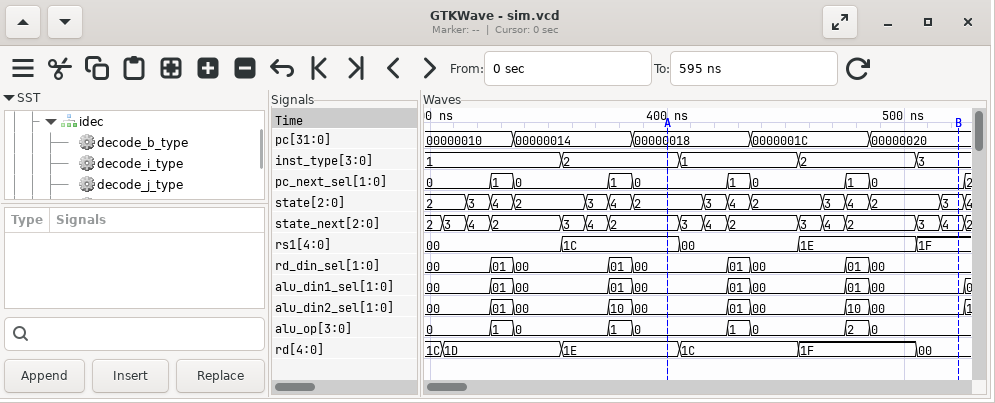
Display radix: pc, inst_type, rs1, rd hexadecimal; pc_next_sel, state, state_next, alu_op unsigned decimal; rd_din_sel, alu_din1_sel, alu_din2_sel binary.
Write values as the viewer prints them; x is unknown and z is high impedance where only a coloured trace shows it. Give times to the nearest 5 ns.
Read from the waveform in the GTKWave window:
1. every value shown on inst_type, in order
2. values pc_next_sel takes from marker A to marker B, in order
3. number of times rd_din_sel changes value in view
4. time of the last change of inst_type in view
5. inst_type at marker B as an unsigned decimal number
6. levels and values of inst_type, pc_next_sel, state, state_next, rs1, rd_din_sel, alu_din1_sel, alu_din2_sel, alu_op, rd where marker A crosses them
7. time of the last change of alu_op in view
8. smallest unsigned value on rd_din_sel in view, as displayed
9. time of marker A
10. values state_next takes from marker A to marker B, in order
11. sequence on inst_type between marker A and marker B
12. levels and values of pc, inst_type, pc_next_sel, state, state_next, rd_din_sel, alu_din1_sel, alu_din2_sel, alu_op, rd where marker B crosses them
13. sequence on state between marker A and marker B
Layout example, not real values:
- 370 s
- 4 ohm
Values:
- 1, 2, 1, 2, 3
- 0, 1, 0, 1, 0
- 8
- 505 ns
- 3
- inst_type=2, pc_next_sel=0, state=2, state_next=2, rs1=1C, rd_din_sel=00, alu_din1_sel=00, alu_din2_sel=00, alu_op=0, rd=1E
- 485 ns
- 00
- 400 ns
- 2, 3, 4, 2, 3, 4, 2, 3, 4
- 2, 1, 2, 3
- pc=00000020, inst_type=3, pc_next_sel=0, state=3, state_next=4, rd_din_sel=00, alu_din1_sel=00, alu_din2_sel=00, alu_op=0, rd=00
- 2, 3, 4, 2, 3, 4, 2, 3
